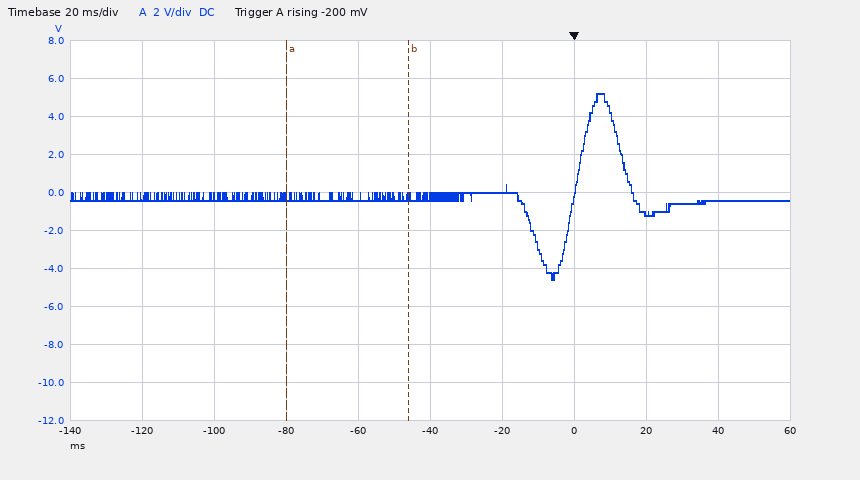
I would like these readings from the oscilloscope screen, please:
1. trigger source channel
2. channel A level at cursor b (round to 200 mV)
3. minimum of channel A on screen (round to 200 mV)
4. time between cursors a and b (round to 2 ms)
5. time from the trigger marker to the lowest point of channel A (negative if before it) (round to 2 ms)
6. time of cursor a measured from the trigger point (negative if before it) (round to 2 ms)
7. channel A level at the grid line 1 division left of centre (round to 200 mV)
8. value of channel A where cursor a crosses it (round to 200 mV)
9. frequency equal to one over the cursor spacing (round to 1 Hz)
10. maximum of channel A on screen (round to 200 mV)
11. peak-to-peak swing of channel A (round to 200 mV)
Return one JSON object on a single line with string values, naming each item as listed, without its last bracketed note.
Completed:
{"trigger source channel": "channel A", "channel A level at cursor b": "-200 mV", "minimum of channel A on screen": "-4.6 V", "time between cursors a and b": "34 ms", "time from the trigger marker to the lowest point of channel A (negative if before it)": "-6 ms", "time of cursor a measured from the trigger point (negative if before it)": "-80 ms", "channel A level at the grid line 1 division left of centre": "-200 mV", "value of channel A where cursor a crosses it": "-200 mV", "frequency equal to one over the cursor spacing": "29 Hz", "maximum of channel A on screen": "5.2 V", "peak-to-peak swing of channel A": "9.8 V"}
